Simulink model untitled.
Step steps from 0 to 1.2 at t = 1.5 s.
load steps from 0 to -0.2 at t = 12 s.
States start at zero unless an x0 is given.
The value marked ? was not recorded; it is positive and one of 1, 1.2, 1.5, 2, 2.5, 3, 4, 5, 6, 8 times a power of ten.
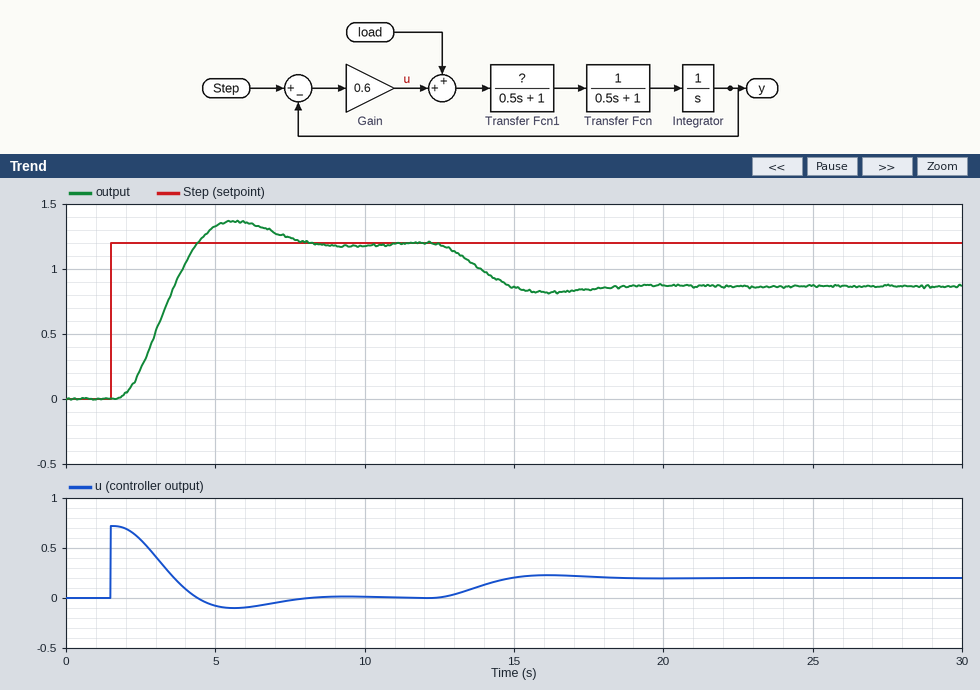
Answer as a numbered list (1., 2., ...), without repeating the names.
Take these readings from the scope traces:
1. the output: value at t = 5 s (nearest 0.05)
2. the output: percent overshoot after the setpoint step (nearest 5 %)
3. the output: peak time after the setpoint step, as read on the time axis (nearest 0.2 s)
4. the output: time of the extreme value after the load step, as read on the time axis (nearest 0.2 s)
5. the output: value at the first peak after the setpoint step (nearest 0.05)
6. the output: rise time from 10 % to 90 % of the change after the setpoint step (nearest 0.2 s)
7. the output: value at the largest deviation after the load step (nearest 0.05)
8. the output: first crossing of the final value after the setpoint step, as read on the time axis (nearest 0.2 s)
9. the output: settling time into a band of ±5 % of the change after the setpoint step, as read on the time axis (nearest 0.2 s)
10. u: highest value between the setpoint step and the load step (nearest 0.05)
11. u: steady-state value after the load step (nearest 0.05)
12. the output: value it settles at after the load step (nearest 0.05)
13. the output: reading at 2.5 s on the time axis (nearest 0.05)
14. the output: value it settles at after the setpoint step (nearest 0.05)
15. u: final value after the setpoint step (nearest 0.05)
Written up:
1. 1.35
2. 15 %
3. 5.6 s
4. 16.2 s
5. 1.35
6. 1.8 s
7. 0.80
8. 4.4 s
9. 7.2 s
10. 0.70
11. 0.20
12. 0.85
13. 0.25
14. 1.20
15. 0.00
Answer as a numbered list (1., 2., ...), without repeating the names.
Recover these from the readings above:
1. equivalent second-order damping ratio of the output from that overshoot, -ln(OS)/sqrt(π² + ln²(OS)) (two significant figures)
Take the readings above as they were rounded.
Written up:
1. 0.52
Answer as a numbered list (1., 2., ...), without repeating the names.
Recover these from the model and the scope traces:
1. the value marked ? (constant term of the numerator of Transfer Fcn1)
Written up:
1. 1.2
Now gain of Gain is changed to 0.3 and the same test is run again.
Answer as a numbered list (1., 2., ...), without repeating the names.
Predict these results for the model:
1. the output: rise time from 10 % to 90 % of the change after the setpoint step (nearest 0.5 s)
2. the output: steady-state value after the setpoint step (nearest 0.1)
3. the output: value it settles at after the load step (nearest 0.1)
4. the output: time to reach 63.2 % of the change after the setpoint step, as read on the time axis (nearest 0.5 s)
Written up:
1. 4.0 s
2. 1.2
3. 0.5
4. 4.5 s
